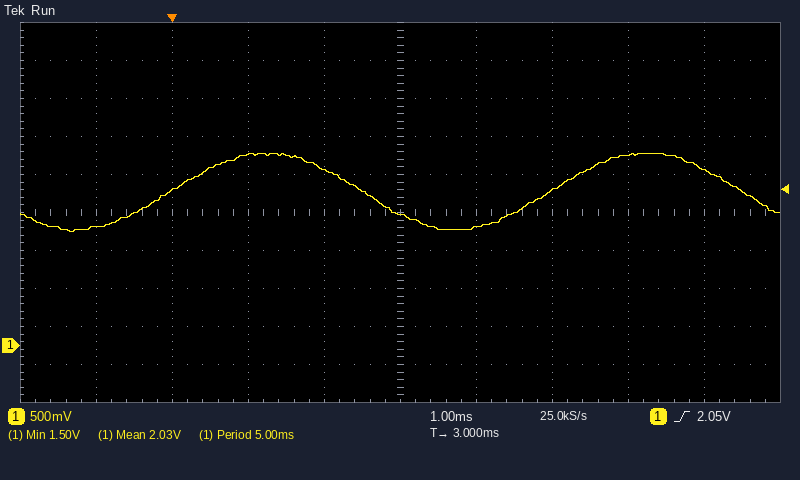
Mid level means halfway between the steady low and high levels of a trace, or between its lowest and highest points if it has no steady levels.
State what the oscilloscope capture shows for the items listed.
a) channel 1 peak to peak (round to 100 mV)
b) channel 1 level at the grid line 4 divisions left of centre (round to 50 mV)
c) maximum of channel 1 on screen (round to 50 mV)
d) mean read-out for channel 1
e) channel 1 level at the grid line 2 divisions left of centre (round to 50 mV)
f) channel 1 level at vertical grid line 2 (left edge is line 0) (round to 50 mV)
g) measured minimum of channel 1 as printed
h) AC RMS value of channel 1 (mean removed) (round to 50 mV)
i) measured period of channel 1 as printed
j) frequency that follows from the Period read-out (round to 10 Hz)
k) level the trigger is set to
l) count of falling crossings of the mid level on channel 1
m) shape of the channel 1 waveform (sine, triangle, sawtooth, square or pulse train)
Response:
1.00 V
1.55 V
2.55 V
2.03 V
2.50 V
2.05 V
1.50 V
350 mV
5.00 ms
200 Hz
2.05 V
2
sine
